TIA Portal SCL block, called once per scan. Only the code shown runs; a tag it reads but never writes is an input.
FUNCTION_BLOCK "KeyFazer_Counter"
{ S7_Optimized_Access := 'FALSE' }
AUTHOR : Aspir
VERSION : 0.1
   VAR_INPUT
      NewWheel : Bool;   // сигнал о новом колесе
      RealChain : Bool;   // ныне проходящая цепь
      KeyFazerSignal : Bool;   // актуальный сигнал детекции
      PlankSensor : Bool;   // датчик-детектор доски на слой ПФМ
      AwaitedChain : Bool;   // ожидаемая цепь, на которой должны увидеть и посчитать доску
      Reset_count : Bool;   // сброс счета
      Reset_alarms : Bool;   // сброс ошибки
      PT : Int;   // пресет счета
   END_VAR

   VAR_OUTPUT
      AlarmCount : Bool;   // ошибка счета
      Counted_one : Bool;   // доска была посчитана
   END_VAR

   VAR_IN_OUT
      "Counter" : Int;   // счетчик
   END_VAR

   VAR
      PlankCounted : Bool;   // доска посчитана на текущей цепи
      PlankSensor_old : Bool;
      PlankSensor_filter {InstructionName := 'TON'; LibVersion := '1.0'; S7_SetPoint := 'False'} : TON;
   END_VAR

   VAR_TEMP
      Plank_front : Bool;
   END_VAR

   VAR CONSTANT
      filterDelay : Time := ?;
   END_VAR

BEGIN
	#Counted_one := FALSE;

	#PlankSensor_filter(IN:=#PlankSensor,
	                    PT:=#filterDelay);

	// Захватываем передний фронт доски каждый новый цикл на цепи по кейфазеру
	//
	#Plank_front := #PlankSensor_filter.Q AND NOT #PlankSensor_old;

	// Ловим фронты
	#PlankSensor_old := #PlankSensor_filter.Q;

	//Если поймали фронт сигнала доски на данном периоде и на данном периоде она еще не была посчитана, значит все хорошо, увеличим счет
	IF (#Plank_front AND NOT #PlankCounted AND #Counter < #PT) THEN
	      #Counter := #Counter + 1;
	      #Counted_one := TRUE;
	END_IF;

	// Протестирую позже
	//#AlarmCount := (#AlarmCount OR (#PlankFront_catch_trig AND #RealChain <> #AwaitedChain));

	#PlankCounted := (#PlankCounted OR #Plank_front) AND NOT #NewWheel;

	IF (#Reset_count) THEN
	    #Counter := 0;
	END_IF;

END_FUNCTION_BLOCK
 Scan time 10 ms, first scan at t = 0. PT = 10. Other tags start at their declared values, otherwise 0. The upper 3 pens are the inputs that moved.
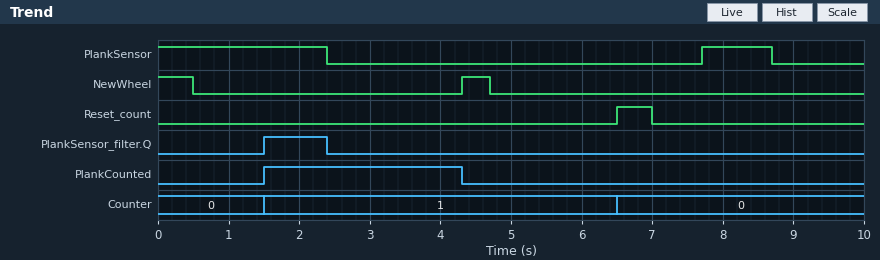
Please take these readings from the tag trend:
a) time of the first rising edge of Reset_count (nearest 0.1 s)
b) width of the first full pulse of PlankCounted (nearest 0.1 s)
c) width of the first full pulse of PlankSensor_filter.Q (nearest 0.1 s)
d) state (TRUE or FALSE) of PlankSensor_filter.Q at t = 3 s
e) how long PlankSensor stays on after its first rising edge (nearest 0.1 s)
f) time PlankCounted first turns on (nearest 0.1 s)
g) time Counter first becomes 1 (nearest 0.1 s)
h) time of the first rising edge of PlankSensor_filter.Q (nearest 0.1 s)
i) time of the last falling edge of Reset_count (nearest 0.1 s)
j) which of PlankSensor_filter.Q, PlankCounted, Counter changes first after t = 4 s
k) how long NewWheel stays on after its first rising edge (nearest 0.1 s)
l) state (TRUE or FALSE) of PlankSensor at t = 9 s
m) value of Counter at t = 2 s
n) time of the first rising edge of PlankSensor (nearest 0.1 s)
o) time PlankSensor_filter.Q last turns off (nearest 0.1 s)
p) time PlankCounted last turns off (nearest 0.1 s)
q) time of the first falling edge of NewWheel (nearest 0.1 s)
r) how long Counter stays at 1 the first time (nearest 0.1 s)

6.5 s
2.8 s
0.9 s
FALSE
1.0 s
1.5 s
1.5 s
1.5 s
7.0 s
PlankCounted
0.4 s
FALSE
1
7.7 s
2.4 s
4.3 s
0.5 s
5.0 s
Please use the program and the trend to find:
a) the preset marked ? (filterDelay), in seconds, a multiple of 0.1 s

1.5 s
